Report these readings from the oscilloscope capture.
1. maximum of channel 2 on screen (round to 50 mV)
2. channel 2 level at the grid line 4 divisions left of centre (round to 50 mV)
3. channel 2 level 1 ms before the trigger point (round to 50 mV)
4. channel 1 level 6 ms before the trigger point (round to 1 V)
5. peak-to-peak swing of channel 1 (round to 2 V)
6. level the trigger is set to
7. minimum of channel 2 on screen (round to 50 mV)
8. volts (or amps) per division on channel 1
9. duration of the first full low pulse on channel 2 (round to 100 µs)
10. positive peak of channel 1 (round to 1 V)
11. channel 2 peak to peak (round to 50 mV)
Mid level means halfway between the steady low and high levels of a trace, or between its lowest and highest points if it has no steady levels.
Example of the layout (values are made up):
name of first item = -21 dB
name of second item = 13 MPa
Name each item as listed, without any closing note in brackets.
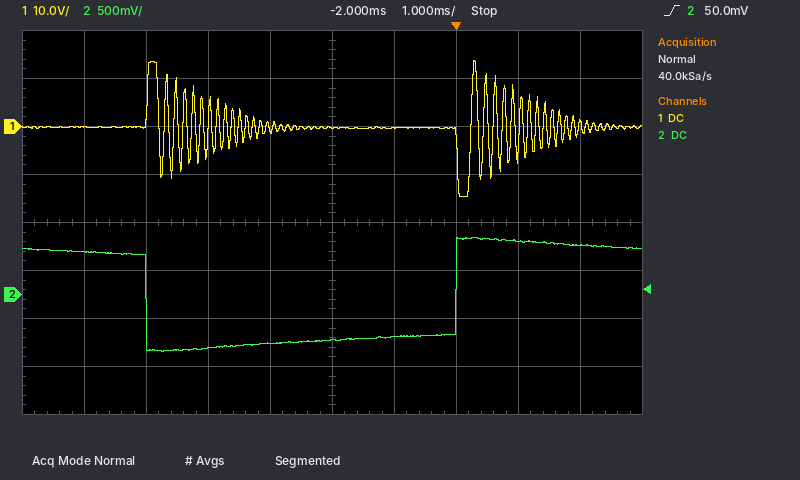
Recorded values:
maximum of channel 2 on screen = 600 mV
channel 2 level at the grid line 4 divisions left of centre = 450 mV
channel 2 level 1 ms before the trigger point = -450 mV
channel 1 level 6 ms before the trigger point = 0 V
peak-to-peak swing of channel 1 = 28 V
level the trigger is set to = 50.0 mV
minimum of channel 2 on screen = -600 mV
volts (or amps) per division on channel 1 = 10 V
duration of the first full low pulse on channel 2 = 5.0 ms
positive peak of channel 1 = 14 V
channel 2 peak to peak = 1.20 V
